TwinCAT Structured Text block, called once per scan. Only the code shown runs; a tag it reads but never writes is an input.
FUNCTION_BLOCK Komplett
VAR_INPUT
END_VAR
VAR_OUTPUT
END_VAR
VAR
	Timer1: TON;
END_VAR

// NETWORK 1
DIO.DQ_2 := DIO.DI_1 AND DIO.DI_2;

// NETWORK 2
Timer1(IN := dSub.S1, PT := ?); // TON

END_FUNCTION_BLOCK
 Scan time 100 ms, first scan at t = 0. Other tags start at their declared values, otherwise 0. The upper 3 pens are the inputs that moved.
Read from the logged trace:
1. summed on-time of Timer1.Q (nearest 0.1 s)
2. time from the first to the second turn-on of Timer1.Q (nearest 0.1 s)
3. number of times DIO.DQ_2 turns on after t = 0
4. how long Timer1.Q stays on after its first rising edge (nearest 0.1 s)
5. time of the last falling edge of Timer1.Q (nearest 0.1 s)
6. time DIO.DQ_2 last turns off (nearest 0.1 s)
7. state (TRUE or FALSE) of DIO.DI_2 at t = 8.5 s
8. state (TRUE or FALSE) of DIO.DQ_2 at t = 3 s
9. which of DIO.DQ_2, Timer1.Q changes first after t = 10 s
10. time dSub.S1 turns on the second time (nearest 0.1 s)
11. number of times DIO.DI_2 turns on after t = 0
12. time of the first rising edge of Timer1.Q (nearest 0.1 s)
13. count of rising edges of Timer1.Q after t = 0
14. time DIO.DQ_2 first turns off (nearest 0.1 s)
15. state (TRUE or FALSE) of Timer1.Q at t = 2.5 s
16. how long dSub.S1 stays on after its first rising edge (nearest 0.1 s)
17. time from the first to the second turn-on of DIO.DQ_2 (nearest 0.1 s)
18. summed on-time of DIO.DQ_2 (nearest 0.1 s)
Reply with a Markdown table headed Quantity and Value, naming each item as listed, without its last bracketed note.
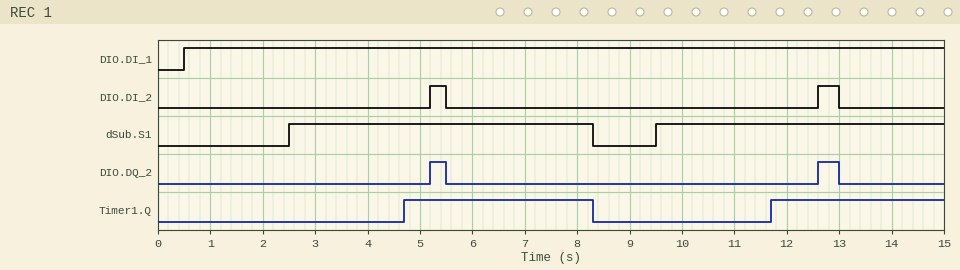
| Quantity | Value |
|---|---|
| summed on-time of Timer1.Q | 6.9 s |
| time from the first to the second turn-on of Timer1.Q | 7.0 s |
| number of times DIO.DQ_2 turns on after t = 0 | 2 |
| how long Timer1.Q stays on after its first rising edge | 3.6 s |
| time of the last falling edge of Timer1.Q | 8.3 s |
| time DIO.DQ_2 last turns off | 13.0 s |
| state (TRUE or FALSE) of DIO.DI_2 at t = 8.5 s | FALSE |
| state (TRUE or FALSE) of DIO.DQ_2 at t = 3 s | FALSE |
| which of DIO.DQ_2, Timer1.Q changes first after t = 10 s | Timer1.Q |
| time dSub.S1 turns on the second time | 9.5 s |
| number of times DIO.DI_2 turns on after t = 0 | 2 |
| time of the first rising edge of Timer1.Q | 4.7 s |
| count of rising edges of Timer1.Q after t = 0 | 2 |
| time DIO.DQ_2 first turns off | 5.5 s |
| state (TRUE or FALSE) of Timer1.Q at t = 2.5 s | FALSE |
| how long dSub.S1 stays on after its first rising edge | 5.8 s |
| time from the first to the second turn-on of DIO.DQ_2 | 7.4 s |
| summed on-time of DIO.DQ_2 | 0.7 s |
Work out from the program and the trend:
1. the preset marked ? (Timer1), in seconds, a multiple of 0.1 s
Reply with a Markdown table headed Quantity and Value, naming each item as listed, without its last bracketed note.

| Quantity | Value |
|---|---|
| the preset marked ? (Timer1), in seconds, a multiple of 0.1 s | 2.2 s |
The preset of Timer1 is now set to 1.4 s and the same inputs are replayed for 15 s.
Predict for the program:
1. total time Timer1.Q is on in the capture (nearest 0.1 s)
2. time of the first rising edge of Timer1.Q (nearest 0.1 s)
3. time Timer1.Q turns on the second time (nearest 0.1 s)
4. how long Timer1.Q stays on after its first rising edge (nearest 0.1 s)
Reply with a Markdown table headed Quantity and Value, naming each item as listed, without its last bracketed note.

| Quantity | Value |
|---|---|
| total time Timer1.Q is on in the capture | 8.5 s |
| time of the first rising edge of Timer1.Q | 3.9 s |
| time Timer1.Q turns on the second time | 10.9 s |
| how long Timer1.Q stays on after its first rising edge | 4.4 s |
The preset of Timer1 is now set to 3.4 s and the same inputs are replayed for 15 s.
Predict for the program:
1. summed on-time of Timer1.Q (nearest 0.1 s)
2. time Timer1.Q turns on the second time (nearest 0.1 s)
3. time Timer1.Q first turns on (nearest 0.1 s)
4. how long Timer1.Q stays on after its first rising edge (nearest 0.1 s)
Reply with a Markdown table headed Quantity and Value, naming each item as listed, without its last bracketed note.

| Quantity | Value |
|---|---|
| summed on-time of Timer1.Q | 4.5 s |
| time Timer1.Q turns on the second time | 12.9 s |
| time Timer1.Q first turns on | 5.9 s |
| how long Timer1.Q stays on after its first rising edge | 2.4 s |
